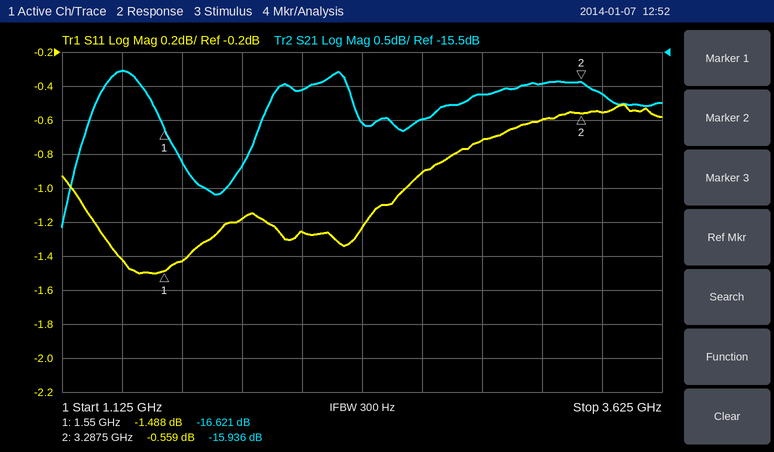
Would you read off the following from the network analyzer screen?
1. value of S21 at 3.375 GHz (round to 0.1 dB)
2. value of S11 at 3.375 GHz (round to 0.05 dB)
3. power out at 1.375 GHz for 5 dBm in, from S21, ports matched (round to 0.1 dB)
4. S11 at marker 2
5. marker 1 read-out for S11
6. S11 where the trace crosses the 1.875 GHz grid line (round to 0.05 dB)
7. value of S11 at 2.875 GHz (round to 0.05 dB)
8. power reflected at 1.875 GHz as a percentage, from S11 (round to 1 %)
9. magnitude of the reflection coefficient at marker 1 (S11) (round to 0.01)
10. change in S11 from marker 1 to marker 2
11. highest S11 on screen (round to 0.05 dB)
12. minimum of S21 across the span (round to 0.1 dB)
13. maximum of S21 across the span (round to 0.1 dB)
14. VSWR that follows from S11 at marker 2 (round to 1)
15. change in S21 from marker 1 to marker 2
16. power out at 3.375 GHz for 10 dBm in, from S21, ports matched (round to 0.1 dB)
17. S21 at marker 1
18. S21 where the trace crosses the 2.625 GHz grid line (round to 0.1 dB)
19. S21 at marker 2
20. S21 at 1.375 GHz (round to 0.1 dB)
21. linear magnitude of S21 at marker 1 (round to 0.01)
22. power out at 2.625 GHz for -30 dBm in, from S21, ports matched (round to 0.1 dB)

-16.1 dB
-0.55 dB
-10.8 dBm
-0.559 dB
-1.488 dB
-1.20 dB
-0.70 dB
76 %
0.84
0.929 dB
-0.50 dB
-18.1 dB
-15.8 dB
31
0.685 dB
-6.1 dBm
-16.621 dB
-16.5 dB
-15.936 dB
-15.8 dB
0.15
-46.5 dBm
